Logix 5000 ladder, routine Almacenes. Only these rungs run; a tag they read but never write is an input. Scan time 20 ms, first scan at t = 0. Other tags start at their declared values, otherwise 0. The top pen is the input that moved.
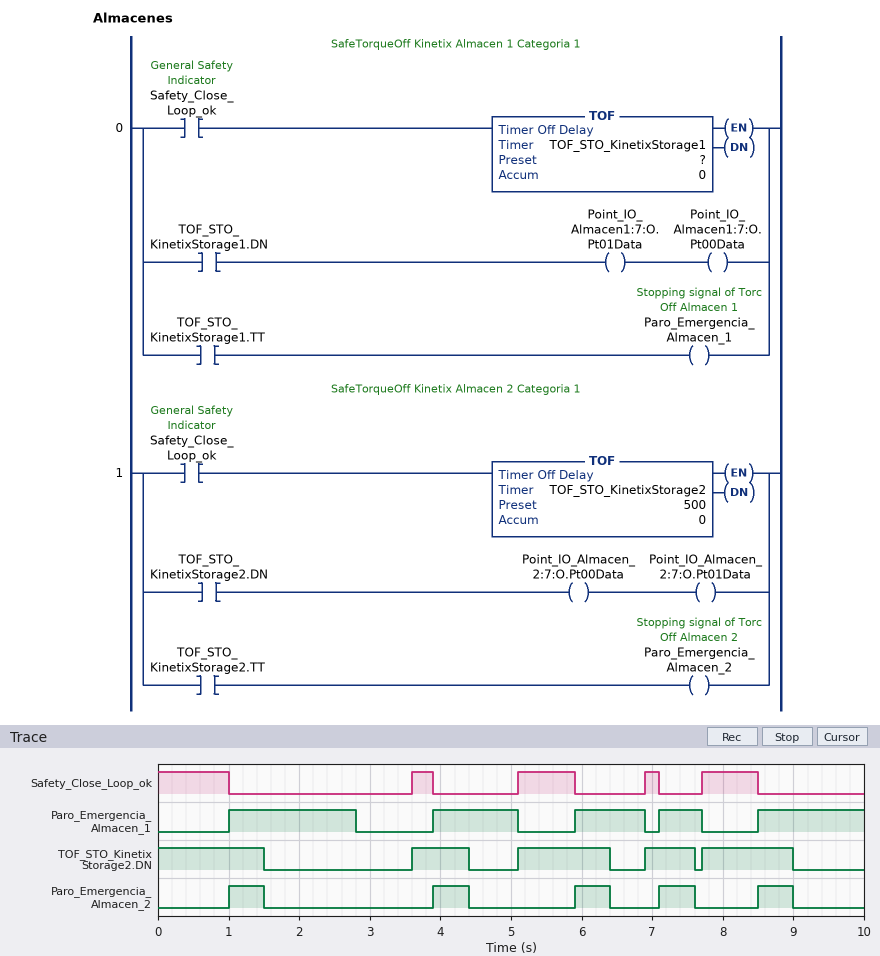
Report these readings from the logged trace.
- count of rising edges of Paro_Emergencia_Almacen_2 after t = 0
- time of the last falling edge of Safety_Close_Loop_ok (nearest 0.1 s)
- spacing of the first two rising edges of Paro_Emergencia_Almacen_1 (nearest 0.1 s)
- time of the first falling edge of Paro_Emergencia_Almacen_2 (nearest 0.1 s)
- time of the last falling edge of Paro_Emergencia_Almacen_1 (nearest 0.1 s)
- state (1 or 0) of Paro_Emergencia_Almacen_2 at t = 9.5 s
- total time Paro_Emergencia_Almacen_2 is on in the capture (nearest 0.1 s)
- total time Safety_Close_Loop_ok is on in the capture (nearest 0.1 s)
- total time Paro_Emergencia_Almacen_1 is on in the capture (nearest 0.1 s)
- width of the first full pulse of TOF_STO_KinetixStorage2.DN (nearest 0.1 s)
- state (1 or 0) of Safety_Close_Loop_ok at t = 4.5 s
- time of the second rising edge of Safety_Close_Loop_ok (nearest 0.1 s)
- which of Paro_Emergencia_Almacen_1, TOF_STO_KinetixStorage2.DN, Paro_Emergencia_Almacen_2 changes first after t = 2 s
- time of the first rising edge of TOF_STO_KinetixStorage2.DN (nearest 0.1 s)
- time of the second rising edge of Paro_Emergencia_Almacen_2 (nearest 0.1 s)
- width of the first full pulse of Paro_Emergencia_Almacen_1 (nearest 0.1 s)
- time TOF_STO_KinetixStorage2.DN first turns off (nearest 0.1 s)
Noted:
5
8.5 s
2.9 s
1.5 s
7.7 s
0
2.5 s
3.1 s
6.1 s
0.8 s
0
5.1 s
Paro_Emergencia_Almacen_1
3.6 s
3.9 s
1.8 s
1.5 s
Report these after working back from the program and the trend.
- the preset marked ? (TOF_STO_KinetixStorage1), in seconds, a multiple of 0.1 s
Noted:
1.8 s
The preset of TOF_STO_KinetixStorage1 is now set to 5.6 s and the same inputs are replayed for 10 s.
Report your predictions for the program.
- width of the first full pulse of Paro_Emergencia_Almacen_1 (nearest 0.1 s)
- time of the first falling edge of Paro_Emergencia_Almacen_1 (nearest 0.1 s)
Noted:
2.6 s
3.6 s
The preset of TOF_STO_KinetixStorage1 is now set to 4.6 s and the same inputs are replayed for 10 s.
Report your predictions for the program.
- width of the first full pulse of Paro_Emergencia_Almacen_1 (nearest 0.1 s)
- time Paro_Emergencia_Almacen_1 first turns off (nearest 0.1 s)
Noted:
2.6 s
3.6 s
